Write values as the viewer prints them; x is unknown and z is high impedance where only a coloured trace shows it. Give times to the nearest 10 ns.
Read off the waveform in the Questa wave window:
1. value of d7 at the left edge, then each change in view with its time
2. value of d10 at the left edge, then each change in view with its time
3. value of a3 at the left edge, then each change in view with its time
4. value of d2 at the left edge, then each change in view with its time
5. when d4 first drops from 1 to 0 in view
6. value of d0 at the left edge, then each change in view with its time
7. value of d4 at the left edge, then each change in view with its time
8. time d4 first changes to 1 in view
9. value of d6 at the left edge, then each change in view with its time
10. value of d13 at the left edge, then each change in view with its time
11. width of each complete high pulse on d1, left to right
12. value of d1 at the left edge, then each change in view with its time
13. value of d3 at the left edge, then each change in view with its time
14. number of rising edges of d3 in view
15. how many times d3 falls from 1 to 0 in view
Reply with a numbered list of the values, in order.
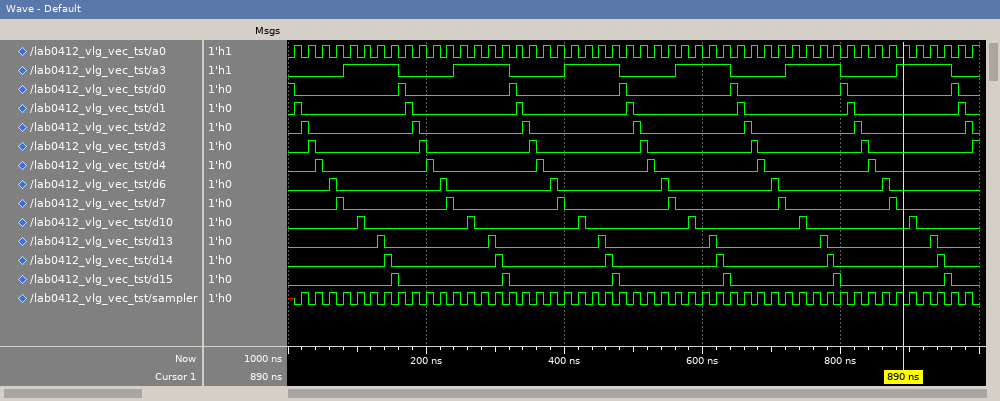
1. 0, 1 at 70 ns, 0 at 80 ns, 1 at 230 ns, 0 at 240 ns, 1 at 390 ns, 0 at 400 ns, 1 at 550 ns, 0 at 560 ns, 1 at 710 ns, 0 at 720 ns, 1 at 870 ns, 0 at 880 ns
2. 0, 1 at 100 ns, 0 at 110 ns, 1 at 260 ns, 0 at 270 ns, 1 at 420 ns, 0 at 430 ns, 1 at 580 ns, 0 at 590 ns, 1 at 740 ns, 0 at 750 ns, 1 at 900 ns, 0 at 910 ns
3. 0, 1 at 80 ns, 0 at 160 ns, 1 at 240 ns, 0 at 320 ns, 1 at 400 ns, 0 at 480 ns, 1 at 560 ns, 0 at 640 ns, 1 at 720 ns, 0 at 800 ns, 1 at 880 ns, 0 at 960 ns
4. 0, 1 at 20 ns, 0 at 30 ns, 1 at 180 ns, 0 at 190 ns, 1 at 340 ns, 0 at 350 ns, 1 at 500 ns, 0 at 510 ns, 1 at 660 ns, 0 at 670 ns, 1 at 820 ns, 0 at 830 ns, 1 at 980 ns, 0 at 990 ns
5. 50 ns
6. 1, 0 at 10 ns, 1 at 160 ns, 0 at 170 ns, 1 at 320 ns, 0 at 330 ns, 1 at 480 ns, 0 at 490 ns, 1 at 640 ns, 0 at 650 ns, 1 at 800 ns, 0 at 810 ns, 1 at 960 ns, 0 at 970 ns
7. 0, 1 at 40 ns, 0 at 50 ns, 1 at 200 ns, 0 at 210 ns, 1 at 360 ns, 0 at 370 ns, 1 at 520 ns, 0 at 530 ns, 1 at 680 ns, 0 at 690 ns, 1 at 840 ns, 0 at 850 ns
8. 40 ns
9. 0, 1 at 60 ns, 0 at 70 ns, 1 at 220 ns, 0 at 230 ns, 1 at 380 ns, 0 at 390 ns, 1 at 540 ns, 0 at 550 ns, 1 at 700 ns, 0 at 710 ns, 1 at 860 ns, 0 at 870 ns
10. 0, 1 at 130 ns, 0 at 140 ns, 1 at 290 ns, 0 at 300 ns, 1 at 450 ns, 0 at 460 ns, 1 at 610 ns, 0 at 620 ns, 1 at 770 ns, 0 at 780 ns, 1 at 930 ns, 0 at 940 ns
11. 10 ns, 10 ns, 10 ns, 10 ns, 10 ns, 10 ns, 10 ns
12. 0, 1 at 10 ns, 0 at 20 ns, 1 at 170 ns, 0 at 180 ns, 1 at 330 ns, 0 at 340 ns, 1 at 490 ns, 0 at 500 ns, 1 at 650 ns, 0 at 660 ns, 1 at 810 ns, 0 at 820 ns, 1 at 970 ns, 0 at 980 ns
13. 0, 1 at 30 ns, 0 at 40 ns, 1 at 190 ns, 0 at 200 ns, 1 at 350 ns, 0 at 360 ns, 1 at 510 ns, 0 at 520 ns, 1 at 670 ns, 0 at 680 ns, 1 at 830 ns, 0 at 840 ns, 1 at 990 ns
14. 7
15. 6
